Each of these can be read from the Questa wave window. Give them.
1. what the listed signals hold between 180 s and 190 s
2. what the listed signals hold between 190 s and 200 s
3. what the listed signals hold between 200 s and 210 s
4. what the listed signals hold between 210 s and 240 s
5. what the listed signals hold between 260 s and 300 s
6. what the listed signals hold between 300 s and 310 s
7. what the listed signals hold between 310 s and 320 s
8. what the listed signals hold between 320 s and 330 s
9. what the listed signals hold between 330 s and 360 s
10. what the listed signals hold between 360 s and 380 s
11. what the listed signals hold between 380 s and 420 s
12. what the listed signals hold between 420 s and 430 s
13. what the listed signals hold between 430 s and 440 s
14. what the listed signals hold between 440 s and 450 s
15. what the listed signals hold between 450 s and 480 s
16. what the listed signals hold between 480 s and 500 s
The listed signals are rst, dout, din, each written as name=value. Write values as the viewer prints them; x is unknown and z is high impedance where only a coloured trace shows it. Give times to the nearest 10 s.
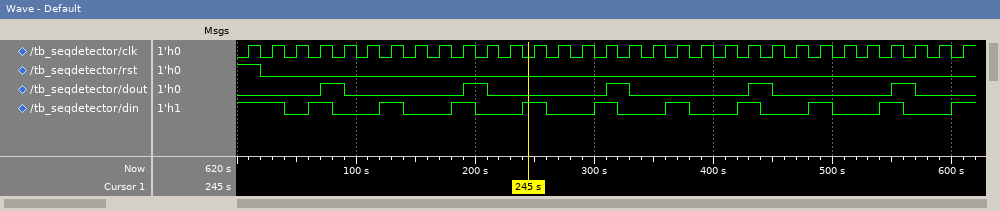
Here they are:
rst=0, dout=0, din=1
rst=0, dout=1, din=1
rst=0, dout=1, din=0
rst=0, dout=0, din=0
rst=0, dout=0, din=0
rst=0, dout=0, din=1
rst=0, dout=1, din=1
rst=0, dout=1, din=0
rst=0, dout=0, din=0
rst=0, dout=0, din=1
rst=0, dout=0, din=0
rst=0, dout=0, din=1
rst=0, dout=1, din=1
rst=0, dout=1, din=0
rst=0, dout=0, din=0
rst=0, dout=0, din=1
